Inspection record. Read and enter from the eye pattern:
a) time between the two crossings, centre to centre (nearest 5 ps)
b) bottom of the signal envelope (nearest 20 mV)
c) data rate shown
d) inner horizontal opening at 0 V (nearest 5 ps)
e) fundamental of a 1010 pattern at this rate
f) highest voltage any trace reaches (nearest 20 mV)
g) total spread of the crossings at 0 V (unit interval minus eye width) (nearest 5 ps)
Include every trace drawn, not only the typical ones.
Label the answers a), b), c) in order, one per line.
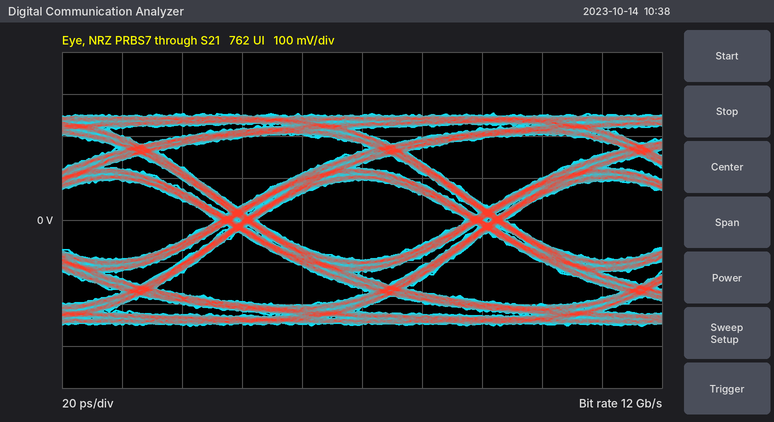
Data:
a) 85 ps
b) -260 mV
c) 12 Gb/s
d) 70 ps
e) 6 GHz
f) 260 mV
g) 15 ps
